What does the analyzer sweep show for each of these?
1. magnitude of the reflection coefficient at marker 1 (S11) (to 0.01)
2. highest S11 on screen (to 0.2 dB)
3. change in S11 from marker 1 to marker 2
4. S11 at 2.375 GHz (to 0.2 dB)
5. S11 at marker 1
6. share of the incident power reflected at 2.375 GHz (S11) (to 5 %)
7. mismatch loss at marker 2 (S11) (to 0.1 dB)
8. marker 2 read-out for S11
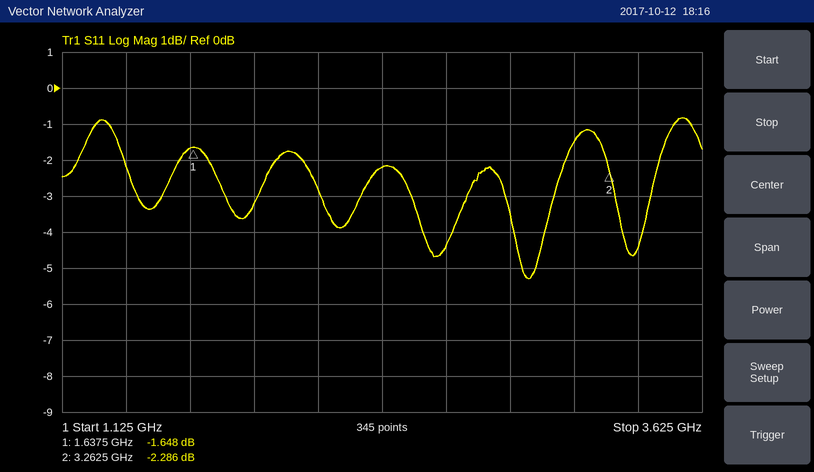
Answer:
0.83
-0.8 dB
-0.638 dB
-2.2 dB
-1.648 dB
60 %
3.9 dB
-2.286 dB
